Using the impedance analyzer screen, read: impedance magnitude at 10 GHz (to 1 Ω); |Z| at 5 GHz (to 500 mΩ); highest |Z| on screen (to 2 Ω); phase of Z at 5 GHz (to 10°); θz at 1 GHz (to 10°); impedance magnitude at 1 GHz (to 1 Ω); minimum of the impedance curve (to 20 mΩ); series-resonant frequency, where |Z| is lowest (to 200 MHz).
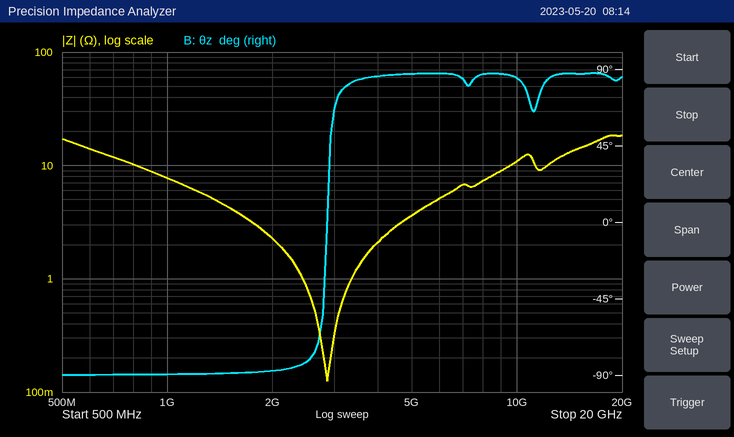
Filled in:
11 Ω
3.5 Ω
18 Ω
90°
-90°
8 Ω
120 mΩ
2.8 GHz
